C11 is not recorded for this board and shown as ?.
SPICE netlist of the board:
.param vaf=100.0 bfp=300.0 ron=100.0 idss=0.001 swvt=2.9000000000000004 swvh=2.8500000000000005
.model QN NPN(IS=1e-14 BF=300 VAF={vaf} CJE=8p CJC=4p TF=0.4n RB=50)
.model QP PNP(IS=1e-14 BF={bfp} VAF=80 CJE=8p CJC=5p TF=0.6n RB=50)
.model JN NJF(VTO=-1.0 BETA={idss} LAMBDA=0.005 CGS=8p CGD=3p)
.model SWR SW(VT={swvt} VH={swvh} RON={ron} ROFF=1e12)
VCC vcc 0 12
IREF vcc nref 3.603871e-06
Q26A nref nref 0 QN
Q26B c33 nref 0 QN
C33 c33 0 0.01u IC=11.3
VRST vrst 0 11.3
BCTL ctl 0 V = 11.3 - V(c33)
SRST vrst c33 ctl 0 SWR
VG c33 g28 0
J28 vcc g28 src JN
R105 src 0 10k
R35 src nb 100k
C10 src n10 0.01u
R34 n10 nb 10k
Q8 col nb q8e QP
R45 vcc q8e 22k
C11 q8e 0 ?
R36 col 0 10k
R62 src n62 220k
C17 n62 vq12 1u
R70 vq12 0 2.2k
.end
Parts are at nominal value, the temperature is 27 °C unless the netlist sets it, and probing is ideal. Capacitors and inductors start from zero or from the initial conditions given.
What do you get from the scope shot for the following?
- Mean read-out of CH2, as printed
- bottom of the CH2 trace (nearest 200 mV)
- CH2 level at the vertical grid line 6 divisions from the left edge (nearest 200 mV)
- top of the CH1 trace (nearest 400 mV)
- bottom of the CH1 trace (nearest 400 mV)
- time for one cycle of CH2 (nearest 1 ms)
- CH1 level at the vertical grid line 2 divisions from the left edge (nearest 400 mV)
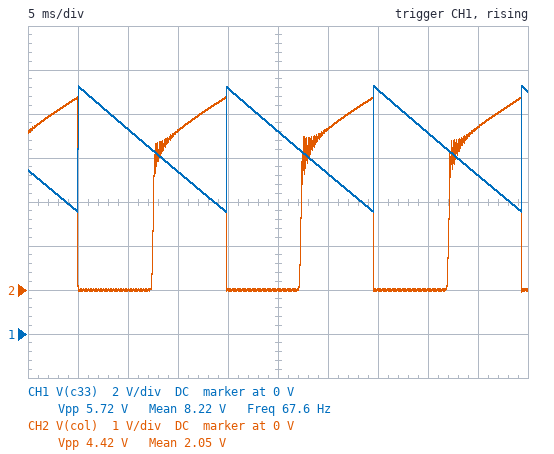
2.05 V
0 V
3.6 V
11.2 V
5.6 V
15 ms
9.2 V
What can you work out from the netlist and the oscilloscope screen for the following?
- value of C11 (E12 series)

560 nF
